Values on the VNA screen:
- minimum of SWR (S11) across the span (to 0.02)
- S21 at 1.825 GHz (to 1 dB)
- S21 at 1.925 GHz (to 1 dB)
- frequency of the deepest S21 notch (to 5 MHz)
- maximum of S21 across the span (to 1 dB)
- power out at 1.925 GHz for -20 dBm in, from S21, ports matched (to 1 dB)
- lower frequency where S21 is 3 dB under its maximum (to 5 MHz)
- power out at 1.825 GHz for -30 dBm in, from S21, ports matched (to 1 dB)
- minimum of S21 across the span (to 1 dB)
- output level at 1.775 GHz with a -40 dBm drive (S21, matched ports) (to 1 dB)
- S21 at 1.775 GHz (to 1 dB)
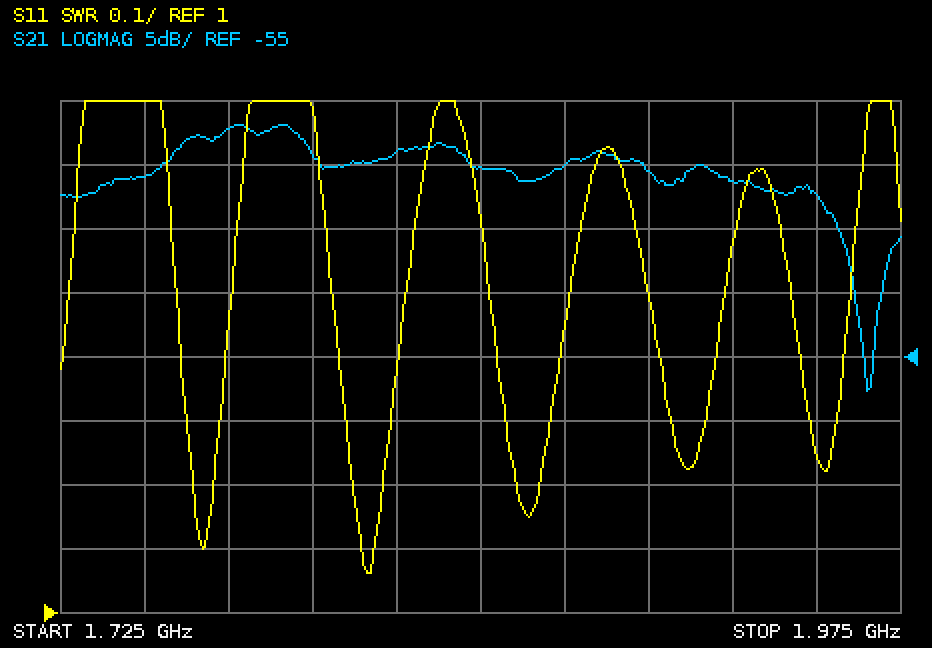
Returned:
1.06
-39 dB
-41 dB
1.965 GHz
-37 dB
-61 dBm
1.755 GHz
-69 dBm
-58 dB
-77 dBm
-37 dB
